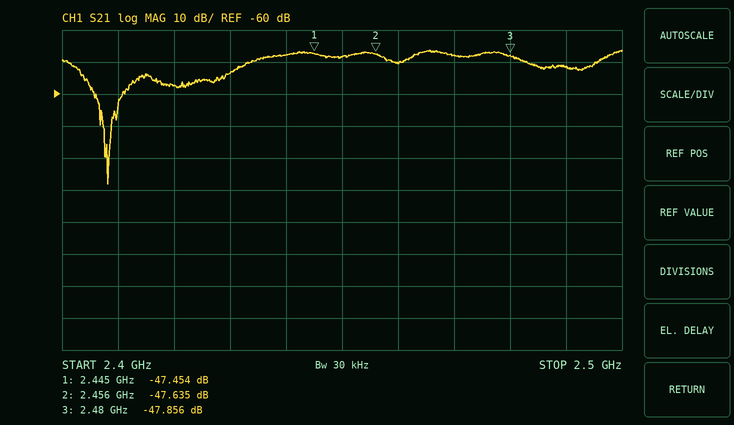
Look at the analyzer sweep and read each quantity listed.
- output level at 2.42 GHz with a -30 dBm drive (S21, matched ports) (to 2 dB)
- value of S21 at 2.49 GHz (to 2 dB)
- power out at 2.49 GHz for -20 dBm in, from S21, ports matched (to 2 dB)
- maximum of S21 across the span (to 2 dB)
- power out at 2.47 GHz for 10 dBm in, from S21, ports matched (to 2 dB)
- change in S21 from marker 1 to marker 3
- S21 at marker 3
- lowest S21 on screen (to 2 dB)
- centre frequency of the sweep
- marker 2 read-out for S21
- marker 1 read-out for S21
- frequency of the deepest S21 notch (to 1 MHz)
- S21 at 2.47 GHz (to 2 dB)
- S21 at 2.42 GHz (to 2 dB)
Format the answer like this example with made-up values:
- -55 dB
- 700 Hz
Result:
- -88 dBm
- -52 dB
- -72 dBm
- -46 dB
- -38 dBm
- -0.402 dB
- -47.856 dB
- -88 dB
- 2.45 GHz
- -47.635 dB
- -47.454 dB
- 2.408 GHz
- -48 dB
- -58 dB
